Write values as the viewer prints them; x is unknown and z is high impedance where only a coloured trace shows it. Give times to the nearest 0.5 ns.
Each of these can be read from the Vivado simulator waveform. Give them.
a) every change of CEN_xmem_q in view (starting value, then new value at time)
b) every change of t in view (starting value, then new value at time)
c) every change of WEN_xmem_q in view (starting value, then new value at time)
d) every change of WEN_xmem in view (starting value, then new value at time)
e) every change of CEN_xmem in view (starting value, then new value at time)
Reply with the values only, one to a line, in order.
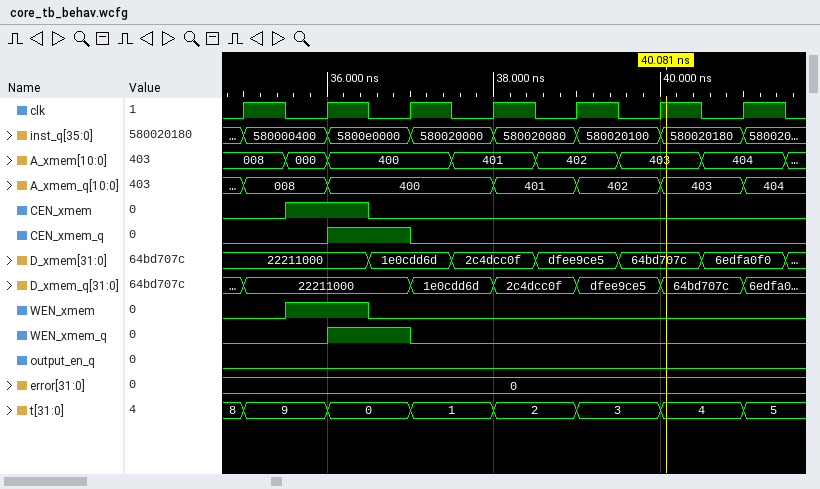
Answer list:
0, 1 at 36 ns, 0 at 37 ns
8, 9 at 35 ns, 0 at 36 ns, 1 at 37 ns, 2 at 38 ns, 3 at 39 ns, 4 at 40 ns, 5 at 41 ns
0, 1 at 36 ns, 0 at 37 ns
0, 1 at 35.5 ns, 0 at 36.5 ns
0, 1 at 35.5 ns, 0 at 36.5 ns
